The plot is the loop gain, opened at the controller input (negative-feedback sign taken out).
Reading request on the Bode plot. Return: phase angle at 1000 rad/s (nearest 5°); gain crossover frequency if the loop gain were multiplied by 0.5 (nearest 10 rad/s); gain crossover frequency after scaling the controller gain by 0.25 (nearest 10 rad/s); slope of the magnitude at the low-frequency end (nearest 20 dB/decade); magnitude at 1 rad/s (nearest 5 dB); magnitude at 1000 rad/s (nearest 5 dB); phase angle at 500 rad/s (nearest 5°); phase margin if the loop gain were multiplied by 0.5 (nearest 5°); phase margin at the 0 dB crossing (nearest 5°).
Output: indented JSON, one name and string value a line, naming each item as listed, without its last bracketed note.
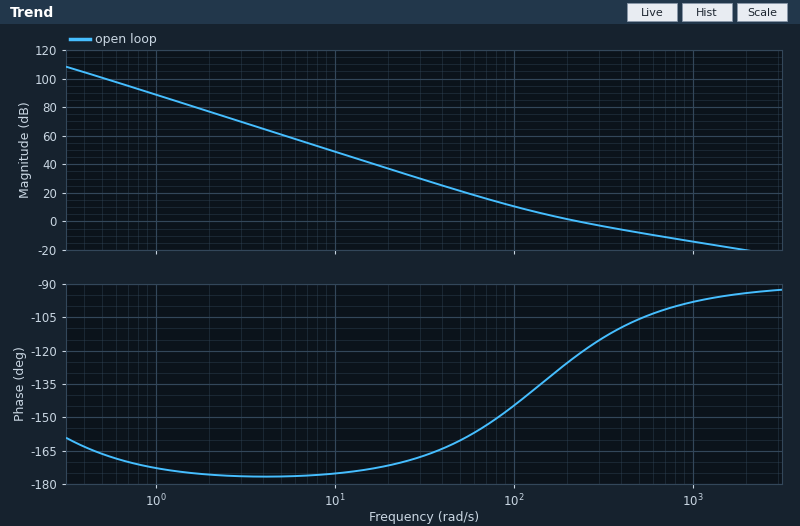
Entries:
{
  "phase angle at 1000 rad/s": "-100°",
  "gain crossover frequency if the loop gain were multiplied by 0.5": "140 rad/s",
  "gain crossover frequency after scaling the controller gain by 0.25": "90 rad/s",
  "slope of the magnitude at the low-frequency end": "-40 dB/decade",
  "magnitude at 1 rad/s": "90 dB",
  "magnitude at 1000 rad/s": "-15 dB",
  "phase angle at 500 rad/s": "-105°",
  "phase margin if the loop gain were multiplied by 0.5": "45°",
  "phase margin at the 0 dB crossing": "60°"
}
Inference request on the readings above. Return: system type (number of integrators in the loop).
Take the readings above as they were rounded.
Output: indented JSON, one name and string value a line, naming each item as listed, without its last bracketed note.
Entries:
{
  "system type": "2"
}
